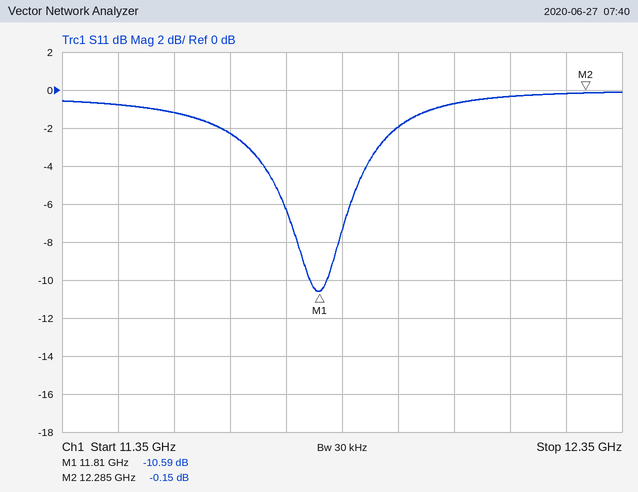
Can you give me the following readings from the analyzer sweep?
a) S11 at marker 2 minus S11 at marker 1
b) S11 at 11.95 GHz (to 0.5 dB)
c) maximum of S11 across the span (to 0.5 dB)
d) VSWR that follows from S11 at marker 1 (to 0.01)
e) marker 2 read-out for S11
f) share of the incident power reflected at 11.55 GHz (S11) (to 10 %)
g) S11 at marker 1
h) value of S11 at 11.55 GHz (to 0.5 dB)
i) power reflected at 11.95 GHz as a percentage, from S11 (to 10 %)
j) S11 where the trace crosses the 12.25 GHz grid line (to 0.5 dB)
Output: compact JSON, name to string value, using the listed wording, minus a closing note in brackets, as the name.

{"S11 at marker 2 minus S11 at marker 1": "10.44 dB", "S11 at 11.95 GHz": "-2.0 dB", "maximum of S11 across the span": "0.0 dB", "VSWR that follows from S11 at marker 1": "1.84", "marker 2 read-out for S11": "-0.15 dB", "share of the incident power reflected at 11.55 GHz (S11)": "80 %", "S11 at marker 1": "-10.59 dB", "value of S11 at 11.55 GHz": "-1.0 dB", "power reflected at 11.95 GHz as a percentage, from S11": "60 %", "S11 where the trace crosses the 12.25 GHz grid line": "0.0 dB"}
